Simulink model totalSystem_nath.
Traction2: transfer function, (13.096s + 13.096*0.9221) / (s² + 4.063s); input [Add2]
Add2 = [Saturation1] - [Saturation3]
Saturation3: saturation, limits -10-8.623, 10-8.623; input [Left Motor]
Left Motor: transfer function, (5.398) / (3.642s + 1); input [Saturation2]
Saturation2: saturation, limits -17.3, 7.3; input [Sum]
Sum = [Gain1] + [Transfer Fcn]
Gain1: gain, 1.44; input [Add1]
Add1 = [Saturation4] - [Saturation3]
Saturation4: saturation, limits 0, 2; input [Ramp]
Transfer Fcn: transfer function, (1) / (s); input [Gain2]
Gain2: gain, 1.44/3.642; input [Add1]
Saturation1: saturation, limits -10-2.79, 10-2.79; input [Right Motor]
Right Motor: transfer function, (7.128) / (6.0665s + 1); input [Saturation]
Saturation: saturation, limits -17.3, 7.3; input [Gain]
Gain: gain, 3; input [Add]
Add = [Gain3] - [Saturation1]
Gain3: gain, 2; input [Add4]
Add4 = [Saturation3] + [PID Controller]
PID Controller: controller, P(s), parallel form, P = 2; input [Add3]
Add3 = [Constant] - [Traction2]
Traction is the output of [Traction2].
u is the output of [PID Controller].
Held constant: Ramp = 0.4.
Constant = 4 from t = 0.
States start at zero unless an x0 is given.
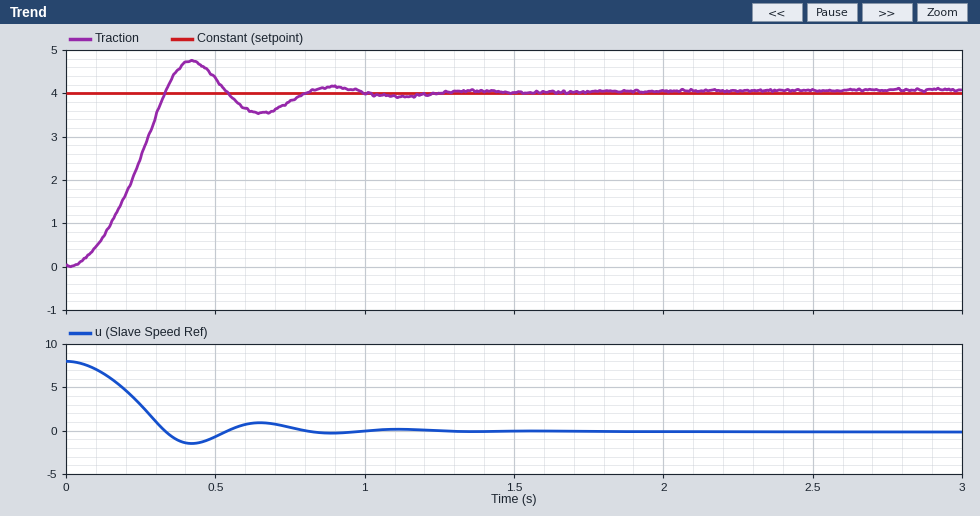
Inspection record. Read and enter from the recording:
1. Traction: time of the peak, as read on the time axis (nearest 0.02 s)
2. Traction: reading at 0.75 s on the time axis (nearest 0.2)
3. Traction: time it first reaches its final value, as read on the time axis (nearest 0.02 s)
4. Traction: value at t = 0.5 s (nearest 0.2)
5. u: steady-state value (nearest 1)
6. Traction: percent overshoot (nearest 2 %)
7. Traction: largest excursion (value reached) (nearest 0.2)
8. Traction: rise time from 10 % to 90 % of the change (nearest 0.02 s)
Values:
0.42 s
3.8
0.34 s
4.4
0
16 %
4.8
0.22 s
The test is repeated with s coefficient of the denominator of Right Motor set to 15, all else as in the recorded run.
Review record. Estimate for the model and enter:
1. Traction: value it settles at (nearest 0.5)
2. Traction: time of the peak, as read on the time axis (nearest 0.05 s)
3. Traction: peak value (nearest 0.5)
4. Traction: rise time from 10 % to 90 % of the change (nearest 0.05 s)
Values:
4.0
0.75 s
4.5
0.40 s
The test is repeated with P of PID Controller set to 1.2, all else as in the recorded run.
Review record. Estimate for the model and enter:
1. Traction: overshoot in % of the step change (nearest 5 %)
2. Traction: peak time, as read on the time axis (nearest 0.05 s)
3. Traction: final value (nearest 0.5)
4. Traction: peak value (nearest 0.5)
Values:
10 %
0.45 s
4.0
4.5
